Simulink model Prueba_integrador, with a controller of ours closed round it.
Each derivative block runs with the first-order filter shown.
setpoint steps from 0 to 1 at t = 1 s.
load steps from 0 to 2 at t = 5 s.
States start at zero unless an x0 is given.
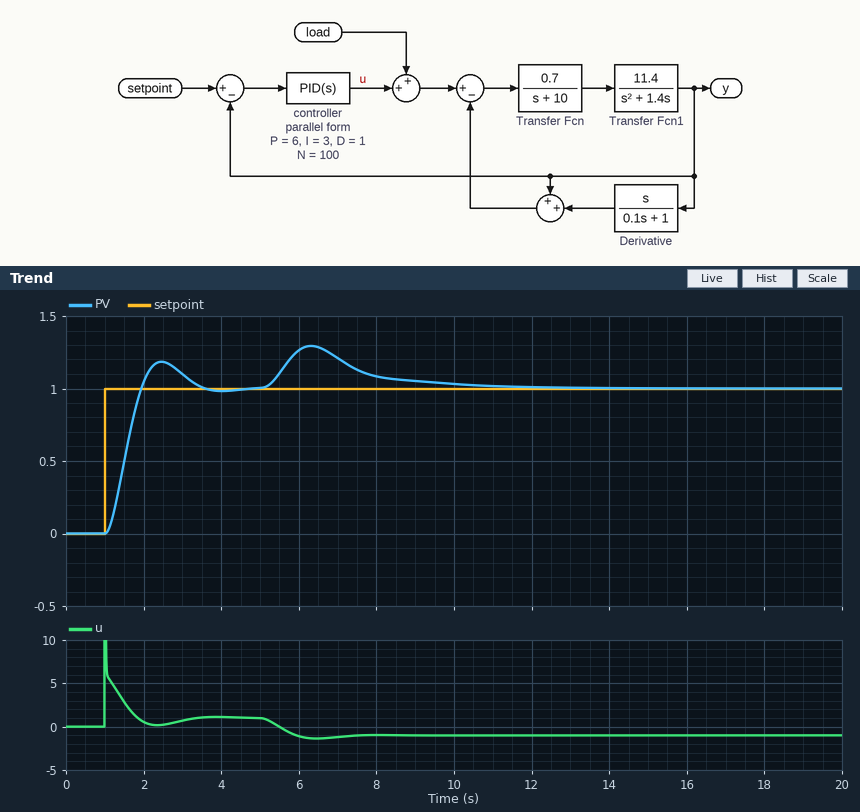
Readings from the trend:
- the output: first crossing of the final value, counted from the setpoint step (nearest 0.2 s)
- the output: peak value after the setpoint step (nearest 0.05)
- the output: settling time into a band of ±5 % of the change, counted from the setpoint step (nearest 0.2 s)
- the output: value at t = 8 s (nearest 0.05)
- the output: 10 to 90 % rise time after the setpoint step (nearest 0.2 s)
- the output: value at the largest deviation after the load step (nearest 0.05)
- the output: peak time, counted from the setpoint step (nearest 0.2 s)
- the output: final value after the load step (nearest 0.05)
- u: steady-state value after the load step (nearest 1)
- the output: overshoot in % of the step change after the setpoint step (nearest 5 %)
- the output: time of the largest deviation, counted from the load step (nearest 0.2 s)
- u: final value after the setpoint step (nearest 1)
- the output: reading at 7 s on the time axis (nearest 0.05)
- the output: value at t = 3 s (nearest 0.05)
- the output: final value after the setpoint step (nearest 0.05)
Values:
1.0 s
1.20
2.2 s
1.10
0.6 s
1.30
1.4 s
1.00
-1
20 %
1.4 s
1
1.20
1.10
1.00
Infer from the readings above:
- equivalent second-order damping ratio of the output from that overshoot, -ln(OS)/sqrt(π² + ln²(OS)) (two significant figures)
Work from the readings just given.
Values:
0.46
